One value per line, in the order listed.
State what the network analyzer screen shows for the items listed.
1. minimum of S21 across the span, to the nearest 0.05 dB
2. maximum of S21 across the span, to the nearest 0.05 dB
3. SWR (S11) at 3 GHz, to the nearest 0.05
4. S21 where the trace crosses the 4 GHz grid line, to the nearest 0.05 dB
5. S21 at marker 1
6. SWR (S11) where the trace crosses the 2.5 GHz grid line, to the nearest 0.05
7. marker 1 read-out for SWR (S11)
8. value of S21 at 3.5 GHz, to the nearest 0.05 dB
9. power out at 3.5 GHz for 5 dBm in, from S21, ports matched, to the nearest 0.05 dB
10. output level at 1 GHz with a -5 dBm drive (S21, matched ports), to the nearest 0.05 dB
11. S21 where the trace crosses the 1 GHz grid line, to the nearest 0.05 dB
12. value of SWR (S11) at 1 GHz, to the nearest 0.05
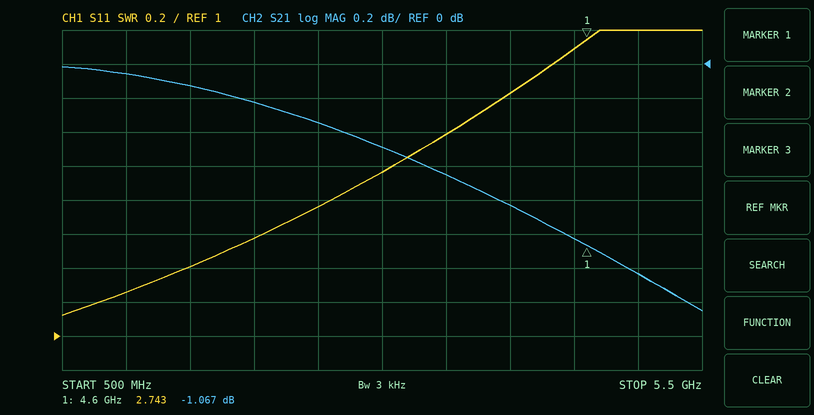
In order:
-1.45 dB
0.00 dB
1.95
-0.85 dB
-1.067 dB
1.75
2.743
-0.65 dB
4.35 dBm
-5.05 dBm
-0.05 dB
1.25
